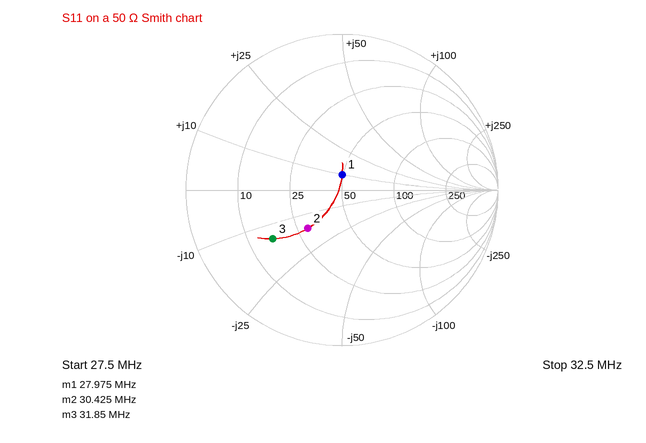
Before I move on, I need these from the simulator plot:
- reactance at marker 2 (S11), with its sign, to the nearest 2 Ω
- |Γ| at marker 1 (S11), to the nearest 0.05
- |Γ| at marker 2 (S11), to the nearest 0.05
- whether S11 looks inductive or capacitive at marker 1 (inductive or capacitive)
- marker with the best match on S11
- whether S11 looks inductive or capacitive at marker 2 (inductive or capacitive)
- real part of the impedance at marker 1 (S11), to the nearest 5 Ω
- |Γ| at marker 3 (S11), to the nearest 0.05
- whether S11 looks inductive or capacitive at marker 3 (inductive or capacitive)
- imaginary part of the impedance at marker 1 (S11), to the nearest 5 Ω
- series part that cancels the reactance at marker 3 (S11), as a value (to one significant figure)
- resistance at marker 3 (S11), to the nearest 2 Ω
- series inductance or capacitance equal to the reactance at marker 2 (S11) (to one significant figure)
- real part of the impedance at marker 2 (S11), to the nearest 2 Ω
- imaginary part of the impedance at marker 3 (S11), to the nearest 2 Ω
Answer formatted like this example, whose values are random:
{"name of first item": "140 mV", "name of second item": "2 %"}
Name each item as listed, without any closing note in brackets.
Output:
{"reactance at marker 2 (S11), with its sign, to the nearest 2 Ω": "-16 Ω", "|Γ| at marker 1 (S11), to the nearest 0.05": "0.10", "|Γ| at marker 2 (S11), to the nearest 0.05": "0.35", "whether S11 looks inductive or capacitive at marker 1": "inductive", "marker with the best match on S11": "marker 1", "whether S11 looks inductive or capacitive at marker 2": "capacitive", "real part of the impedance at marker 1 (S11), to the nearest 5 Ω": "50 Ω", "|Γ| at marker 3 (S11), to the nearest 0.05": "0.55", "whether S11 looks inductive or capacitive at marker 3": "capacitive", "imaginary part of the impedance at marker 1 (S11), to the nearest 5 Ω": "+10 Ω", "series part that cancels the reactance at marker 3 (S11), as a value": "70 nH", "resistance at marker 3 (S11), to the nearest 2 Ω": "16 Ω", "series inductance or capacitance equal to the reactance at marker 2 (S11)": "300 pF", "real part of the impedance at marker 2 (S11), to the nearest 2 Ω": "28 Ω", "imaginary part of the impedance at marker 3 (S11), to the nearest 2 Ω": "-14 Ω"}
